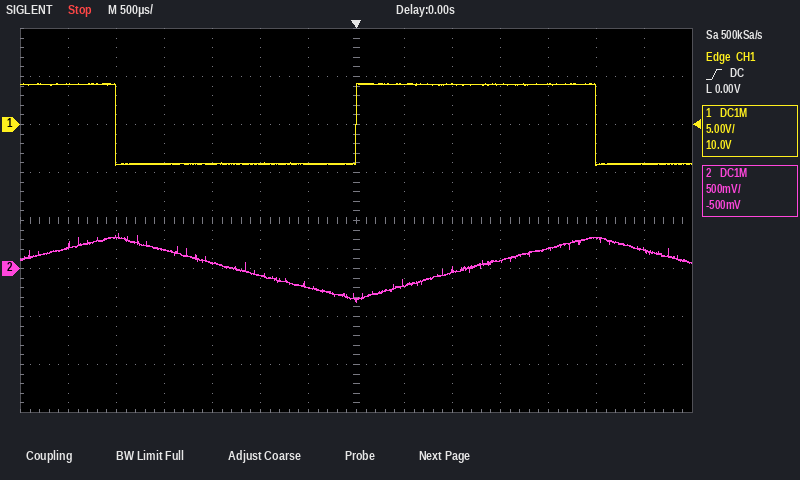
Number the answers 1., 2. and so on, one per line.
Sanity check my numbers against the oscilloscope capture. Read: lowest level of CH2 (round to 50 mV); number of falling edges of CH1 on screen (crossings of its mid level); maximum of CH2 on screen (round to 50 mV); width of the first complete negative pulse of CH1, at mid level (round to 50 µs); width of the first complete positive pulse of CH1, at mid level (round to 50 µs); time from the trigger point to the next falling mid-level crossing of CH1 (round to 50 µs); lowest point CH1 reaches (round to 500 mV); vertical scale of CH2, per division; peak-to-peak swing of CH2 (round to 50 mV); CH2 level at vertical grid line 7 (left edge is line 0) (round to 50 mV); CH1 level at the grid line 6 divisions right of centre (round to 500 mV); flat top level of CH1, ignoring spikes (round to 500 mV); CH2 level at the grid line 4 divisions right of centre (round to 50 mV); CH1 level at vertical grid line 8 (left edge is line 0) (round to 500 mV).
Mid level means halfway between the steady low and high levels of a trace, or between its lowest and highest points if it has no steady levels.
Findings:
1. -350 mV
2. 2
3. 350 mV
4. 2.50 ms
5. 2.50 ms
6. 2.50 ms
7. -4.5 V
8. 500 mV
9. 700 mV
10. -350 mV
11. -4.0 V
12. 4.0 V
13. 200 mV
14. 4.0 V
